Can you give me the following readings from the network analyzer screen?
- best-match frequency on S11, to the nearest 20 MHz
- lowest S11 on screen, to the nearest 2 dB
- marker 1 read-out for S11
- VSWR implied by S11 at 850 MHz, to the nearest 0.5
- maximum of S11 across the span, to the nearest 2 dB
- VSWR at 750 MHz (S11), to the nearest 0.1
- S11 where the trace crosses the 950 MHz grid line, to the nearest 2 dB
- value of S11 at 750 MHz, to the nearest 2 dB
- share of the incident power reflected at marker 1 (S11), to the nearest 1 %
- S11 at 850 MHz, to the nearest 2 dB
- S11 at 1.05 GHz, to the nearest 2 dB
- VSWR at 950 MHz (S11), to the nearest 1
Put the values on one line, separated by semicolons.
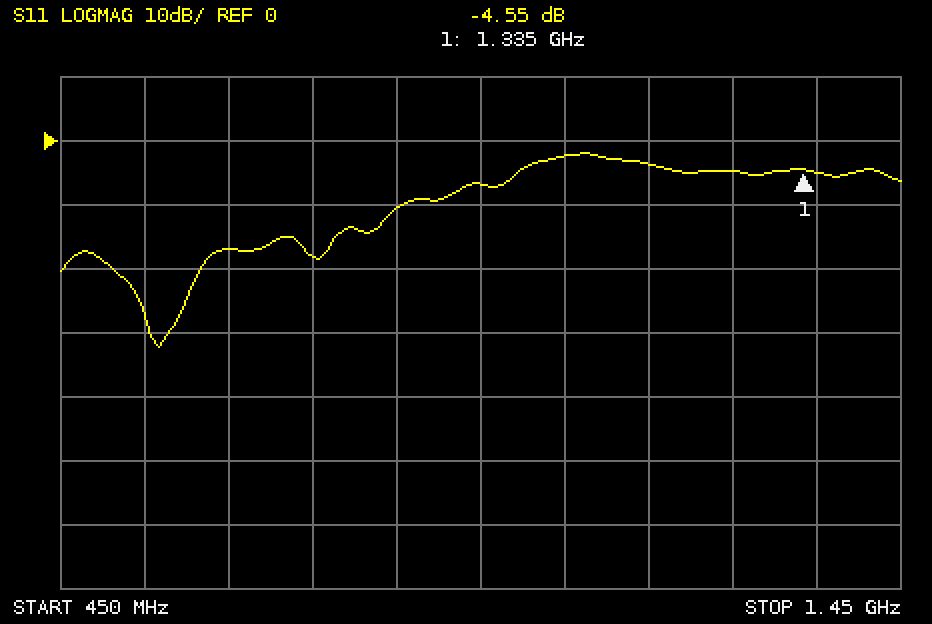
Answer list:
560 MHz; -32 dB; -4.55 dB; 2.0; -2 dB; 1.3; -6 dB; -18 dB; 35 %; -10 dB; -2 dB; 3
